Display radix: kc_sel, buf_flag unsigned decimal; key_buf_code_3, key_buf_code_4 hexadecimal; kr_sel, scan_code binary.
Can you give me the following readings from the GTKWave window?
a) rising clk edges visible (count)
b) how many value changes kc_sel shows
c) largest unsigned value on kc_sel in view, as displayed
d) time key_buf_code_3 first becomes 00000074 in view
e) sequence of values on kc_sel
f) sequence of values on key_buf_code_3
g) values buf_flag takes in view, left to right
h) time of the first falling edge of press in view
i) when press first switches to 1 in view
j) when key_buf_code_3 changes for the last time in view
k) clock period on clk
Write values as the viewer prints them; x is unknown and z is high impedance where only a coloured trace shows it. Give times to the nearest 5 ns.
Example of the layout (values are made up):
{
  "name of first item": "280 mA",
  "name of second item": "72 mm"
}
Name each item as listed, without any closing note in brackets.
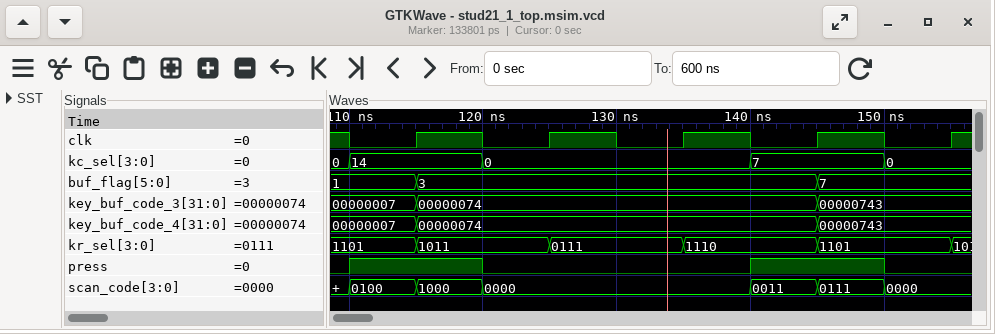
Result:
{
  "rising clk edges visible": "5",
  "how many value changes kc_sel shows": "4",
  "largest unsigned value on kc_sel in view, as displayed": "14",
  "time key_buf_code_3 first becomes 00000074 in view": "115 ns",
  "sequence of values on kc_sel": "0, 14, 0, 7, 0",
  "sequence of values on key_buf_code_3": "00000007, 00000074, 00000743",
  "values buf_flag takes in view, left to right": "1, 3, 7",
  "time of the first falling edge of press in view": "120 ns",
  "when press first switches to 1 in view": "110 ns",
  "when key_buf_code_3 changes for the last time in view": "145 ns",
  "clock period on clk": "10 ns"
}
